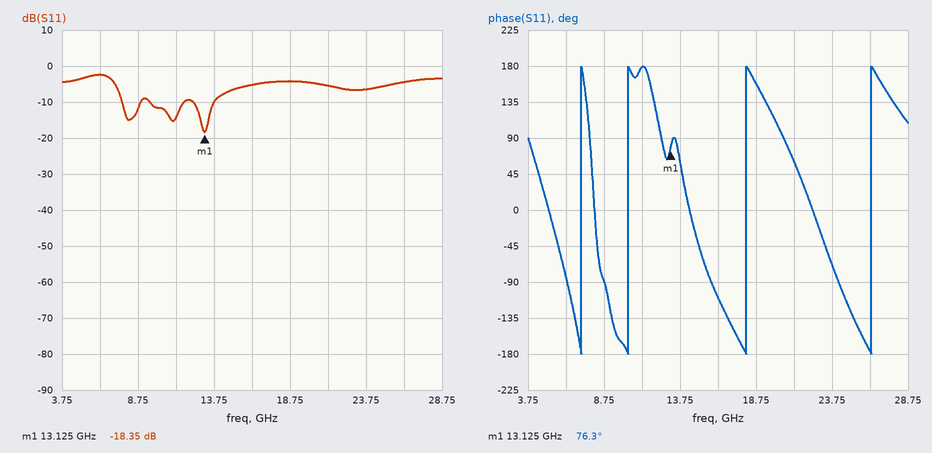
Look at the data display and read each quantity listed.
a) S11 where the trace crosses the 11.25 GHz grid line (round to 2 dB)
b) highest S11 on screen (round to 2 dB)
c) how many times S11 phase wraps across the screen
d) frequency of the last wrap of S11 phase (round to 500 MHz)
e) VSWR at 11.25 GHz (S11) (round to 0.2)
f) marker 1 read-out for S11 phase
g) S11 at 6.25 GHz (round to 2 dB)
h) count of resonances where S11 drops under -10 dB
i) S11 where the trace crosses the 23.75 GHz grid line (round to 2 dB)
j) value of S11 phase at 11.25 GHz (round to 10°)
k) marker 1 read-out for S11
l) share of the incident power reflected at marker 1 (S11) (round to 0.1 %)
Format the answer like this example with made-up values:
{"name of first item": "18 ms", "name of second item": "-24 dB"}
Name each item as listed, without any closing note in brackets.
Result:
{"S11 where the trace crosses the 11.25 GHz grid line": "-14 dB", "highest S11 on screen": "-2 dB", "how many times S11 phase wraps across the screen": "4", "frequency of the last wrap of S11 phase": "26.5 GHz", "VSWR at 11.25 GHz (S11)": "1.4", "marker 1 read-out for S11 phase": "76.3°", "S11 at 6.25 GHz": "-2 dB", "count of resonances where S11 drops under -10 dB": "3", "S11 where the trace crosses the 23.75 GHz grid line": "-6 dB", "value of S11 phase at 11.25 GHz": "180°", "marker 1 read-out for S11": "-18.35 dB", "share of the incident power reflected at marker 1 (S11)": "1.5 %"}
